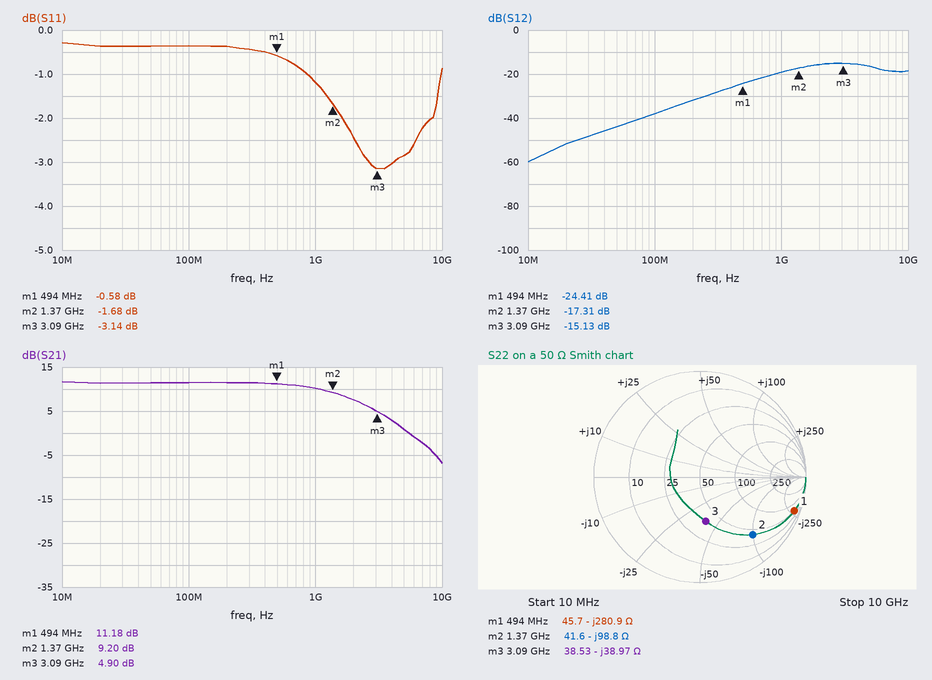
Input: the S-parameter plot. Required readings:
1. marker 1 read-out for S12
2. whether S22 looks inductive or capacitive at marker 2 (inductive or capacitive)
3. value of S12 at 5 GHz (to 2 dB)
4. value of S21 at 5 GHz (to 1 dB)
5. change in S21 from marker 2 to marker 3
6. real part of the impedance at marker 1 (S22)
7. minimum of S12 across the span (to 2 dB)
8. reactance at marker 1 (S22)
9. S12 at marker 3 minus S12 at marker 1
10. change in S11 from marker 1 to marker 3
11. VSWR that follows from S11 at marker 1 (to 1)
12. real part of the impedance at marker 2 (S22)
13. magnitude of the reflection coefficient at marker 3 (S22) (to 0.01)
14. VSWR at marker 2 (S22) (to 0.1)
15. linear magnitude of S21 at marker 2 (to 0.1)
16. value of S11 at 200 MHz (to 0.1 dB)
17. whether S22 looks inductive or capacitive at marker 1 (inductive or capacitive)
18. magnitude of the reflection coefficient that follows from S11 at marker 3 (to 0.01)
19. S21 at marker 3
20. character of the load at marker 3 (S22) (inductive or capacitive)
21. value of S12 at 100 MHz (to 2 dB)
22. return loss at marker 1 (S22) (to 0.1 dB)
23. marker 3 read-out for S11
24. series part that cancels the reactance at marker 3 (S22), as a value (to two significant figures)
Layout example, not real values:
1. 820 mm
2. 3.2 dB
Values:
1. -24.41 dB
2. capacitive
3. -16 dB
4. 1 dB
5. -4.30 dB
6. 45.7 Ω
7. -60 dB
8. -280.9 Ω
9. 9.28 dB
10. -2.56 dB
11. 30
12. 41.6 Ω
13. 0.42
14. 6.6
15. 2.9
16. -0.4 dB
17. capacitive
18. 0.70
19. 4.90 dB
20. capacitive
21. -38 dB
22. 0.5 dB
23. -3.14 dB
24. 2.0 nH
